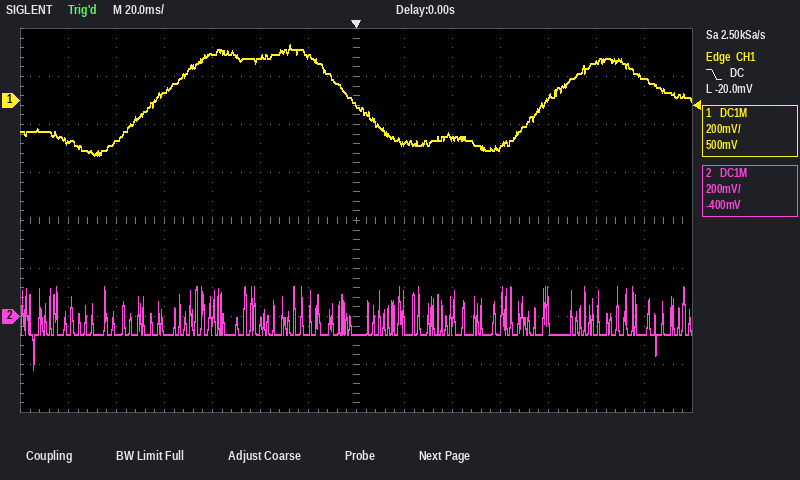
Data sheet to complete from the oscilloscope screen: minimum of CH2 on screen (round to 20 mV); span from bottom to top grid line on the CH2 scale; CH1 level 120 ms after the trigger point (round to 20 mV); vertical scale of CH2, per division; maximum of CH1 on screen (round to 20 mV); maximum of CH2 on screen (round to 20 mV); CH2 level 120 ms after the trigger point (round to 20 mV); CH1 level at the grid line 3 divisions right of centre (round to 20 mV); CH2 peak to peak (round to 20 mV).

-220 mV
1.6 V
100 mV
200 mV
240 mV
120 mV
-80 mV
-200 mV
340 mV
